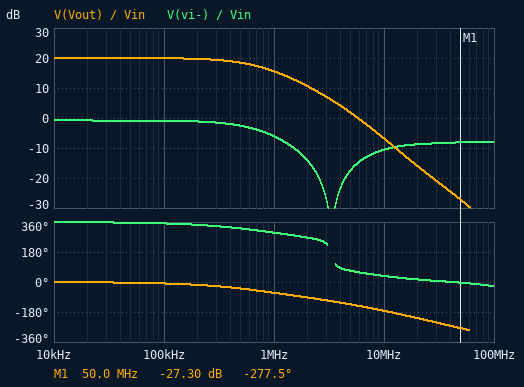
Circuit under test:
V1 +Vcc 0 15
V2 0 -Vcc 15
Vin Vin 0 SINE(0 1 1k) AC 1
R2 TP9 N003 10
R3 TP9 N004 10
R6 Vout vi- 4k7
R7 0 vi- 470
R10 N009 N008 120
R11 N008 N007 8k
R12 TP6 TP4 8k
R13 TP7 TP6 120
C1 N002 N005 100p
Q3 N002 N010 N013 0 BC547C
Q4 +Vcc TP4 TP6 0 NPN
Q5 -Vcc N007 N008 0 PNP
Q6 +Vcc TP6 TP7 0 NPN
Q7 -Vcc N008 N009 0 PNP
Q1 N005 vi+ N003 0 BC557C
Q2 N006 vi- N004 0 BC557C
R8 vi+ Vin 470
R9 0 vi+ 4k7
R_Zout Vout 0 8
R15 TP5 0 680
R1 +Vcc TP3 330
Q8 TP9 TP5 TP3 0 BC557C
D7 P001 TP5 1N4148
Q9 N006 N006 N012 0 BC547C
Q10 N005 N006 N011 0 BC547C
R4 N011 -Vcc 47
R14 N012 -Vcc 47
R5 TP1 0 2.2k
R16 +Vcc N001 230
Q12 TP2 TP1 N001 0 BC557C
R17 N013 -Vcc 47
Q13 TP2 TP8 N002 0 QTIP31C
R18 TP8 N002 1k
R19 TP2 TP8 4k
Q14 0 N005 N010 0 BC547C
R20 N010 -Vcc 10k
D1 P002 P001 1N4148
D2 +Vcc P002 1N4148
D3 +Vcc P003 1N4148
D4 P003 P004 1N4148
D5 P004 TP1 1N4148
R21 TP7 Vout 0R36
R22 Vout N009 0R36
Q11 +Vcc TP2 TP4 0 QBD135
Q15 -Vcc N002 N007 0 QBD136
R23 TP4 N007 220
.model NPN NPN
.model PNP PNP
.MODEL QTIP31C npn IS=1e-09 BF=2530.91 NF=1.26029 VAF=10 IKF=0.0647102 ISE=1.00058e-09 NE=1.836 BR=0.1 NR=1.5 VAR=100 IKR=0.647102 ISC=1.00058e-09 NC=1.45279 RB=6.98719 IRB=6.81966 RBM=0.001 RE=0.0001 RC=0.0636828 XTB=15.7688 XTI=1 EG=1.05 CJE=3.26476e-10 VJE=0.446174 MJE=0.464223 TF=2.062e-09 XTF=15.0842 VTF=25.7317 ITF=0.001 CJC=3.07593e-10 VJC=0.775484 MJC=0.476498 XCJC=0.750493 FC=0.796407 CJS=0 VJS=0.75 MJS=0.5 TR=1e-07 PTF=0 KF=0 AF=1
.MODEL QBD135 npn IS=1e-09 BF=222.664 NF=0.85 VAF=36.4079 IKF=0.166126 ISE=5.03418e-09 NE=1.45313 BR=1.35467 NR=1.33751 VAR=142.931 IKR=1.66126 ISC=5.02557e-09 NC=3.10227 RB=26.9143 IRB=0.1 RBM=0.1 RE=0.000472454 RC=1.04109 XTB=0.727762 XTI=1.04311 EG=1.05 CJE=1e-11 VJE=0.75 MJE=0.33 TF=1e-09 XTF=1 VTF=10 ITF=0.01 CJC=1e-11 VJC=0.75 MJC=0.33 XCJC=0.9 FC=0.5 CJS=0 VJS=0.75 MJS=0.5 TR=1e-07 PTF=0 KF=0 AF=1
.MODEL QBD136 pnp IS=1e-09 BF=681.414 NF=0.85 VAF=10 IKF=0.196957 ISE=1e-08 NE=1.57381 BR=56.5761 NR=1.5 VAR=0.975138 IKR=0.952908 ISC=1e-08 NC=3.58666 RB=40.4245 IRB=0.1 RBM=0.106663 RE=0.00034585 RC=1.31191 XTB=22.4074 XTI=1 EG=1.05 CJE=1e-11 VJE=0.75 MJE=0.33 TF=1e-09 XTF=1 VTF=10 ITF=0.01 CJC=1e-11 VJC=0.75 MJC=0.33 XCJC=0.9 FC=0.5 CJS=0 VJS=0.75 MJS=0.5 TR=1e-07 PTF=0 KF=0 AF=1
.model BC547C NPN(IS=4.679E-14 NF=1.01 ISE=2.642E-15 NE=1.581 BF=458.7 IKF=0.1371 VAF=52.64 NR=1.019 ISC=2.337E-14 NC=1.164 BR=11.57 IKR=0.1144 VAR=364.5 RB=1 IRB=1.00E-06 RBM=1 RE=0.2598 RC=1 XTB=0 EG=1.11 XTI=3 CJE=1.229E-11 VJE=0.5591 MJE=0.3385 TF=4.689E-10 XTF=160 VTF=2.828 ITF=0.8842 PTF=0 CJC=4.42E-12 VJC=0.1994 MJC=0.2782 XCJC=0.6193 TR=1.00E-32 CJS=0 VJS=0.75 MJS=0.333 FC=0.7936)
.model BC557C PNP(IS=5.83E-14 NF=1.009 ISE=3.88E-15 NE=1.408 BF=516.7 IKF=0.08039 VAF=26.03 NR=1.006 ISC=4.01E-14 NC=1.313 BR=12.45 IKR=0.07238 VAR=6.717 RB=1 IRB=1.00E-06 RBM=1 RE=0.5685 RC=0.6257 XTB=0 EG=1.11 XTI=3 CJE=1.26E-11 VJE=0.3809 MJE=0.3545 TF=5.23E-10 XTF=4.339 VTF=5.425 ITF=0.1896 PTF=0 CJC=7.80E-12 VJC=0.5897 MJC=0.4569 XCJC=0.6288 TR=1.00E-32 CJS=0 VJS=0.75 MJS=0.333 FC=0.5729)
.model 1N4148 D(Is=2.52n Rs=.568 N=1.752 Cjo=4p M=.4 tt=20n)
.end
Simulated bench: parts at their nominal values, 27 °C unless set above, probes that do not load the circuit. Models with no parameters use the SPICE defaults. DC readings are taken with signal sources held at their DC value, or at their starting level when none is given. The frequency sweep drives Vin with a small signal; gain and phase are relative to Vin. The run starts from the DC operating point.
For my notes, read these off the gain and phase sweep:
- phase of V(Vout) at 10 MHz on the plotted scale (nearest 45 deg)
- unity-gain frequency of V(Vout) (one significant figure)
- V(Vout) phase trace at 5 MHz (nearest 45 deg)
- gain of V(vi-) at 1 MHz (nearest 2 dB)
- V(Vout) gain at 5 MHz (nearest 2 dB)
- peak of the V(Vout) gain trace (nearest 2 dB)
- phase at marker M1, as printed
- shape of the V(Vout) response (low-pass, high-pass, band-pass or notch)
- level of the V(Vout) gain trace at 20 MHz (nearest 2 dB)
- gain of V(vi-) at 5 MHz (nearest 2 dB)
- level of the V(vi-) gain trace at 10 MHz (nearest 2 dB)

-180 deg
6 MHz
-135 deg
-6 dB
2 dB
20 dB
-277.5 deg
low-pass
-16 dB
-18 dB
-10 dB
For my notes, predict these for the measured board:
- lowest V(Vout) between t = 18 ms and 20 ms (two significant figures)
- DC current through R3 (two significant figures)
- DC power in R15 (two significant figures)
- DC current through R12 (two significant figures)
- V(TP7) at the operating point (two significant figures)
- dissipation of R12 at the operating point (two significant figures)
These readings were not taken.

-10 V
2.3 mA
240 mW
99 µA
5.9 mV
78 µW
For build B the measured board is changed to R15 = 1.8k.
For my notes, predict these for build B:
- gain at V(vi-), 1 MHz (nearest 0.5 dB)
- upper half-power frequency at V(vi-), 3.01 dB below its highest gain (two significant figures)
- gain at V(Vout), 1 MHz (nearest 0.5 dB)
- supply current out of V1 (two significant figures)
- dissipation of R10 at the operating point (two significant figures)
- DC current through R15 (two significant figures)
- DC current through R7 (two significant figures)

-6.5 dB
650 kHz
15.0 dB
34 mA
210 µW
7.2 mA
3.7 µA
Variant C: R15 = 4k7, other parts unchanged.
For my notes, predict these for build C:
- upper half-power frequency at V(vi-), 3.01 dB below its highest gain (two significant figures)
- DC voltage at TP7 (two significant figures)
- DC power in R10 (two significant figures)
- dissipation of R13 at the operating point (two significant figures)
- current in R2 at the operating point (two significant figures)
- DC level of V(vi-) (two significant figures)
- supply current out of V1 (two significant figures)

620 kHz
6.5 mV
210 µW
490 µW
1.9 mA
1.7 mV
29 mA
